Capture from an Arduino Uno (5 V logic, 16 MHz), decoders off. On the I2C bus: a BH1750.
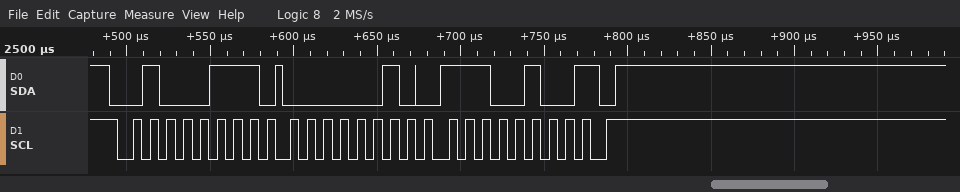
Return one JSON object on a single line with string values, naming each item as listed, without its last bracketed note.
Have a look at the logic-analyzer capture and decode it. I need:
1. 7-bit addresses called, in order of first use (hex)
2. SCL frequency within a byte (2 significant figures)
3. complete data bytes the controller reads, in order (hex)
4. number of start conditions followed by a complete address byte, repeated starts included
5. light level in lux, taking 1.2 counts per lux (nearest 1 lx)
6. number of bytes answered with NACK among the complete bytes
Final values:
{"7-bit addresses called, in order of first use": "0x23", "SCL frequency within a byte": "100 kHz", "complete data bytes the controller reads, in order": "02 E4", "number of start conditions followed by a complete address byte, repeated starts included": "1", "light level in lux, taking 1.2 counts per lux": "617 lx", "number of bytes answered with NACK among the complete bytes": "1"}
